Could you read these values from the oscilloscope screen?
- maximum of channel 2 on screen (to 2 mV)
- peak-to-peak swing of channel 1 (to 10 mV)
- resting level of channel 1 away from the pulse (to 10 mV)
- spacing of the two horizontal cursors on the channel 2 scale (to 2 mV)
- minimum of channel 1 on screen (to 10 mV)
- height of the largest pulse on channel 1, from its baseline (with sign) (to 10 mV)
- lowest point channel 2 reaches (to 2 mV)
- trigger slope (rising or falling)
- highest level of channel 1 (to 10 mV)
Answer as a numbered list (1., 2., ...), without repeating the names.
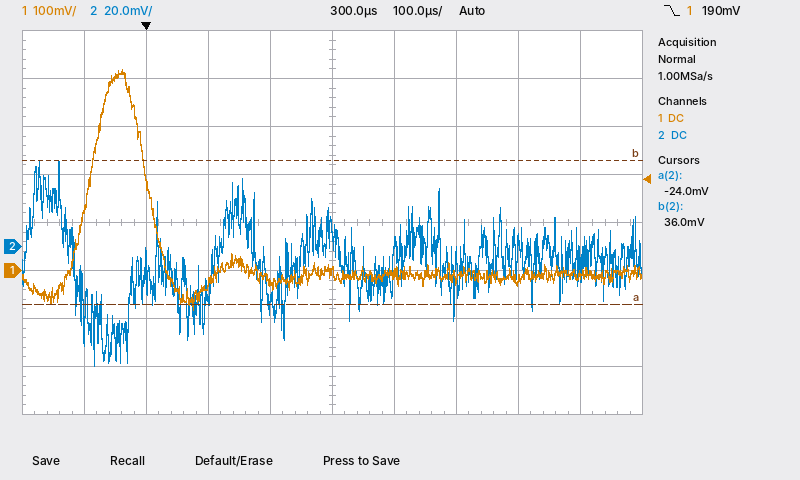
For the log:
1. 36 mV
2. 500 mV
3. -10 mV
4. 60 mV
5. -80 mV
6. +430 mV
7. -50 mV
8. falling
9. 420 mV
